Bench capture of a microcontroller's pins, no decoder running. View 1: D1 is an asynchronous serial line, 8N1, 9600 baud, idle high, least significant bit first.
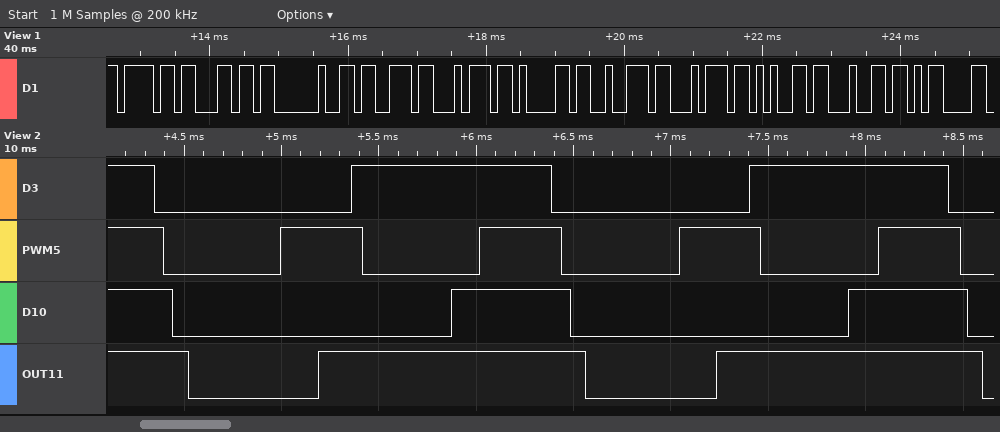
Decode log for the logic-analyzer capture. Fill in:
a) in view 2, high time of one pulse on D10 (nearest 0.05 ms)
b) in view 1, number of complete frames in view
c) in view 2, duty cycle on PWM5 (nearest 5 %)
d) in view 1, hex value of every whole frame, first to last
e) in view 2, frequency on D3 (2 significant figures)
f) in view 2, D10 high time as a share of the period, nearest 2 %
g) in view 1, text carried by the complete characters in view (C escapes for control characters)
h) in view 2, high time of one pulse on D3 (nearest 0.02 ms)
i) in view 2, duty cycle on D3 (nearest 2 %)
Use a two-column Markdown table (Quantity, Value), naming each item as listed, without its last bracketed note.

| Quantity | Value |
|---|---|
| in view 2, high time of one pulse on D10 | 0.60 ms |
| in view 1, number of complete frames in view | 11 |
| in view 2, duty cycle on PWM5 | 40 % |
| in view 1, hex value of every whole frame, first to last | 6F 6C 20 73 74 61 72 74 65 64 0D |
| in view 2, frequency on D3 | 490 Hz |
| in view 2, D10 high time as a share of the period, nearest 2 % | 30 % |
| in view 1, text carried by the complete characters in view | "ol started\r" |
| in view 2, high time of one pulse on D3 | 1.02 ms |
| in view 2, duty cycle on D3 | 50 % |
